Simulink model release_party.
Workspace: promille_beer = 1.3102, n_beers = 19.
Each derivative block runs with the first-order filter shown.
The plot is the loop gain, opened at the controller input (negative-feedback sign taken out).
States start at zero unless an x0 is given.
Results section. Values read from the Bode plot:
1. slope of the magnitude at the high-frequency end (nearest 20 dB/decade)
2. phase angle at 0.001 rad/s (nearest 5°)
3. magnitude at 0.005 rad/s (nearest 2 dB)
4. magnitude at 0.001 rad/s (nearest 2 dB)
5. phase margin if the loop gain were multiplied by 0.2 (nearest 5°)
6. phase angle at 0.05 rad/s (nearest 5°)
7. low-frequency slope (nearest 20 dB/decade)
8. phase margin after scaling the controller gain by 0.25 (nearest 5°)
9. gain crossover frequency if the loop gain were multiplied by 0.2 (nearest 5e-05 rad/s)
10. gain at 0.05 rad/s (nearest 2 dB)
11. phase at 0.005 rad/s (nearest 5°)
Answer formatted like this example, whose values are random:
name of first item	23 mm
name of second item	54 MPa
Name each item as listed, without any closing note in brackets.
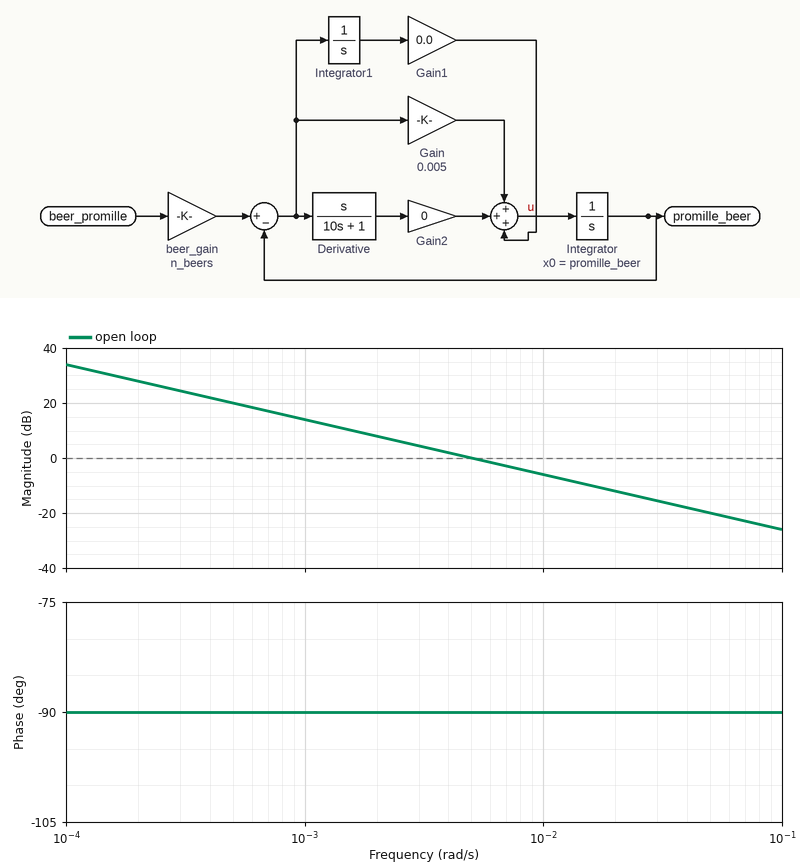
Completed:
slope of the magnitude at the high-frequency end	-20 dB/decade
phase angle at 0.001 rad/s	-90°
magnitude at 0.005 rad/s	0 dB
magnitude at 0.001 rad/s	14 dB
phase margin if the loop gain were multiplied by 0.2	90°
phase angle at 0.05 rad/s	-90°
low-frequency slope	-20 dB/decade
phase margin after scaling the controller gain by 0.25	90°
gain crossover frequency if the loop gain were multiplied by 0.2	0.00100 rad/s
gain at 0.05 rad/s	-20 dB
phase at 0.005 rad/s	-90°
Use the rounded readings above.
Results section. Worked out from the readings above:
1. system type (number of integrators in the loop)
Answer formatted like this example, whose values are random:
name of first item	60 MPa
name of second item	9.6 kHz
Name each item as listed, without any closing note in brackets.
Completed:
system type	1
